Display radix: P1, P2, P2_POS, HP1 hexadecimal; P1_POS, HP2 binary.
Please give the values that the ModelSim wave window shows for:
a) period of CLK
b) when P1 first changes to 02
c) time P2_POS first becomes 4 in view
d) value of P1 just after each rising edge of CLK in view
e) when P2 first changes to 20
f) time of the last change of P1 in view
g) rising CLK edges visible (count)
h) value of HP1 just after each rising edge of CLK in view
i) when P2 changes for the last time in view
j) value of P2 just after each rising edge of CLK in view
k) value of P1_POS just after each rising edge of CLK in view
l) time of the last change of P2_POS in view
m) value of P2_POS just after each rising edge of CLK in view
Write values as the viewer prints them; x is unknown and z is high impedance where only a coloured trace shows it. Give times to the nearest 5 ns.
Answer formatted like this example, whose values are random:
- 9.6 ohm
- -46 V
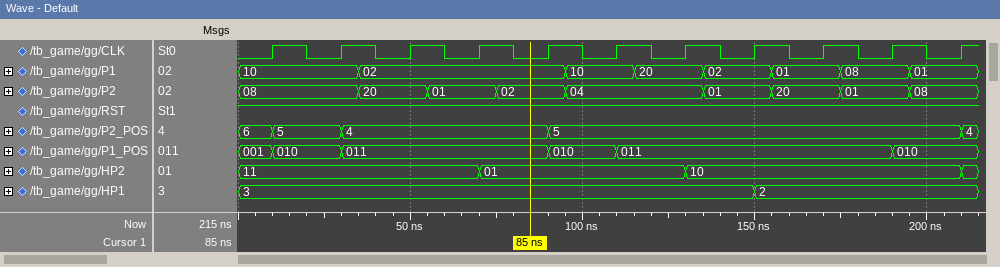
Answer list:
- 20 ns
- 35 ns
- 30 ns
- 10, 10, 02, 02, 02, 10, 20, 02, 01, 08, 01
- 35 ns
- 195 ns
- 11
- 3, 3, 3, 3, 3, 3, 3, 2, 2, 2, 2
- 195 ns
- 08, 08, 20, 01, 02, 04, 04, 01, 20, 01, 08
- 010, 011, 011, 011, 010, 011, 011, 011, 011, 010, 010
- 210 ns
- 5, 4, 4, 4, 5, 5, 5, 5, 5, 5, 4
